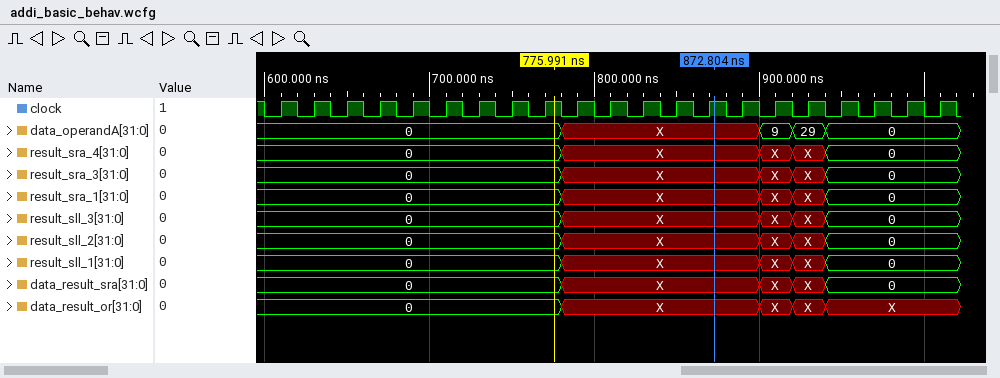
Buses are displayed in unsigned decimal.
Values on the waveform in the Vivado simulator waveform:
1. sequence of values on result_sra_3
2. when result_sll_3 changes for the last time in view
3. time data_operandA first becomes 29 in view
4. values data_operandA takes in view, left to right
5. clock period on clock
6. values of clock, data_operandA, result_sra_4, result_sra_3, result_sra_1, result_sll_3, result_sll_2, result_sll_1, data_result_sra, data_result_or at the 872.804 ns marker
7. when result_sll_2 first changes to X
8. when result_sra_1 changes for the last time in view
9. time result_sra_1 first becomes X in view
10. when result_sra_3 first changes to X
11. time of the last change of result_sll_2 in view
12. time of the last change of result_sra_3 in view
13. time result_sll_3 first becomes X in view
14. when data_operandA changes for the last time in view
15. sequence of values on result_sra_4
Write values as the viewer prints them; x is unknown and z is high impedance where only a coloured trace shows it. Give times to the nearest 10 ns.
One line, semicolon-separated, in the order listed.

0, X, X, X, 0; 940 ns; 920 ns; 0, X, 9, 29, 0; 20 ns; clock=1, data_operandA=X, result_sra_4=X, result_sra_3=X, result_sra_1=X, result_sll_3=X, result_sll_2=X, result_sll_1=X, data_result_sra=X, data_result_or=X; 780 ns; 940 ns; 780 ns; 780 ns; 940 ns; 940 ns; 780 ns; 940 ns; 0, X, X, X, 0
